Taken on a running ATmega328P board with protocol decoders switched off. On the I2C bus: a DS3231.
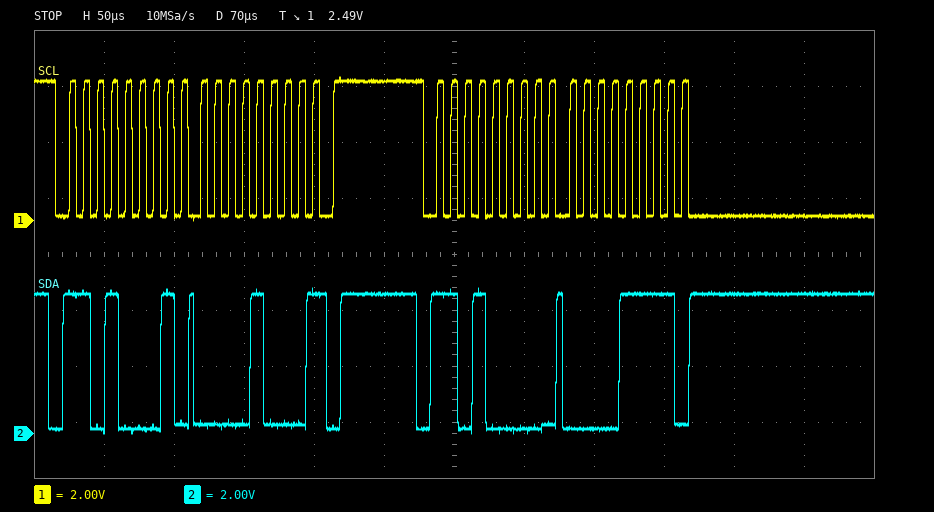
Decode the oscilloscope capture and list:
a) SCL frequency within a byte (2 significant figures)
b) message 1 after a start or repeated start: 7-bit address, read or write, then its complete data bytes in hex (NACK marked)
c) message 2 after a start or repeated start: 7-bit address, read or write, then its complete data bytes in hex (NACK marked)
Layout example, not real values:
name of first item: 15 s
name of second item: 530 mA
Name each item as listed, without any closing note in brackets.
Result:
SCL frequency within a byte: 100 kHz
message 1 after a start or repeated start: 7-bit address, read or write, then its complete data bytes in hex: 0x68 read: 08 NACK
message 2 after a start or repeated start: 7-bit address, read or write, then its complete data bytes in hex: 0x68 write: 0F
